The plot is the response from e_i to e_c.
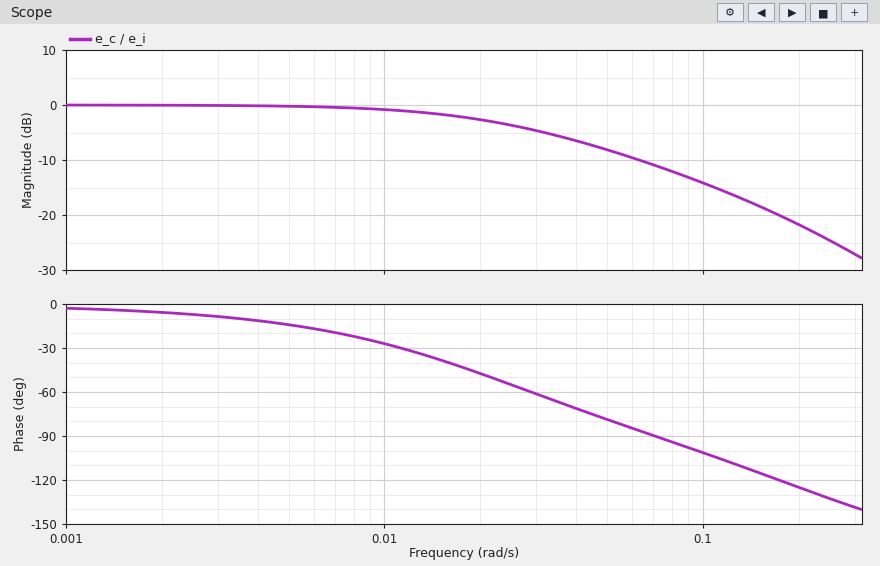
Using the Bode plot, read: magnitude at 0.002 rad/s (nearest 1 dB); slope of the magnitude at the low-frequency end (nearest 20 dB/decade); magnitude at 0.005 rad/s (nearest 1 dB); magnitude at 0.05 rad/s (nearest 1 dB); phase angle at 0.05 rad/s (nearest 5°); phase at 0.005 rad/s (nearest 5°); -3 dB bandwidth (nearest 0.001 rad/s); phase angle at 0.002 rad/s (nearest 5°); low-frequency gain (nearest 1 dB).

0 dB
0 dB/decade
0 dB
-8 dB
-80°
-15°
0.022 rad/s
-5°
0 dB
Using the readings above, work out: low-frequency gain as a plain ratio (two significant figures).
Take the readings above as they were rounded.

1.0
